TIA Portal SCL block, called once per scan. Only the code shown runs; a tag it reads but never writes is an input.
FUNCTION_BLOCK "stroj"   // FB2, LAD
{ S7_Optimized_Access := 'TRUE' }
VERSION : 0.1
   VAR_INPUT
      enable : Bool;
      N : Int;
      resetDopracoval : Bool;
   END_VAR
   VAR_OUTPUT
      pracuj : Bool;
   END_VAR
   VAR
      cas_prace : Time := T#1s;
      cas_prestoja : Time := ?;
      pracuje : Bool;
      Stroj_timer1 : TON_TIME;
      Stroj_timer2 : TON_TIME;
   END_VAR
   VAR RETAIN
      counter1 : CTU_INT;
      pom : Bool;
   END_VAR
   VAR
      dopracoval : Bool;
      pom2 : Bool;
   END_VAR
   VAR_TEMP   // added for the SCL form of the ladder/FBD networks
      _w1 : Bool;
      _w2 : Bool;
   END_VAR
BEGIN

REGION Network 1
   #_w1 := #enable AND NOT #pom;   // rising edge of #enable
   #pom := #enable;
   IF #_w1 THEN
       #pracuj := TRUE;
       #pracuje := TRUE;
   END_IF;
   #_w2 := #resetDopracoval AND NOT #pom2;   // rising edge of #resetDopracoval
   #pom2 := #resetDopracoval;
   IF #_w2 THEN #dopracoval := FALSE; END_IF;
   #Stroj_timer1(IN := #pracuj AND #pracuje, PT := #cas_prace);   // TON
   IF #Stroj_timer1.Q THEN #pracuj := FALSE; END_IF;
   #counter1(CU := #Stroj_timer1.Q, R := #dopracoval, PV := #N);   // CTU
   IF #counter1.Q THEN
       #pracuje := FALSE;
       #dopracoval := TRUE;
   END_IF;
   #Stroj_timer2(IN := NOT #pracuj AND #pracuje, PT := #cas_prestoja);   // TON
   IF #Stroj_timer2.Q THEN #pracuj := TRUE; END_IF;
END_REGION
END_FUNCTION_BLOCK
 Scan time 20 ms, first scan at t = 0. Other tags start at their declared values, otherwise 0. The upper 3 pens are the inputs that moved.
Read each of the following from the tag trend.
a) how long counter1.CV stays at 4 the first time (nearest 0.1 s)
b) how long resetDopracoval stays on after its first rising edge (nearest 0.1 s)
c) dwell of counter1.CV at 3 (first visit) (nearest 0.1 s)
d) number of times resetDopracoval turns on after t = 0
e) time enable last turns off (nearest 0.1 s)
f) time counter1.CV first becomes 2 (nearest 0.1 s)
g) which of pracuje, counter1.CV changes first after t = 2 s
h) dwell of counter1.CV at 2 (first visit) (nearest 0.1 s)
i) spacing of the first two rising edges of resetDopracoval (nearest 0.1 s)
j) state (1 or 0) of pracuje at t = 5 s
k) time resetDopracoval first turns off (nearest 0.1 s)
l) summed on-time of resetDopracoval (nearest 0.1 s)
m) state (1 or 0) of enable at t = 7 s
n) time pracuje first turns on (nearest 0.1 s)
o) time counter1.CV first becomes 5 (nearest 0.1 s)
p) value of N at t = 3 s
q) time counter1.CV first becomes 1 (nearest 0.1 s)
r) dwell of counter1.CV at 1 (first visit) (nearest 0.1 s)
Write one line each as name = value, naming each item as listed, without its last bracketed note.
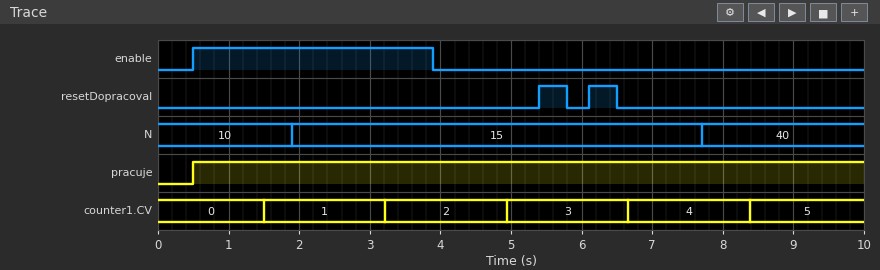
how long counter1.CV stays at 4 the first time = 1.7 s
how long resetDopracoval stays on after its first rising edge = 0.4 s
dwell of counter1.CV at 3 (first visit) = 1.7 s
number of times resetDopracoval turns on after t = 0 = 2
time enable last turns off = 3.9 s
time counter1.CV first becomes 2 = 3.2 s
which of pracuje, counter1.CV changes first after t = 2 s = counter1.CV
dwell of counter1.CV at 2 (first visit) = 1.7 s
spacing of the first two rising edges of resetDopracoval = 0.7 s
state (1 or 0) of pracuje at t = 5 s = 1
time resetDopracoval first turns off = 5.8 s
summed on-time of resetDopracoval = 0.8 s
state (1 or 0) of enable at t = 7 s = 0
time pracuje first turns on = 0.5 s
time counter1.CV first becomes 5 = 8.4 s
value of N at t = 3 s = 15
time counter1.CV first becomes 1 = 1.5 s
dwell of counter1.CV at 1 (first visit) = 1.7 s
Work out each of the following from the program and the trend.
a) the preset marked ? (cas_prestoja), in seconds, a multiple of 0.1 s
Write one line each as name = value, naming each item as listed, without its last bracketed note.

the preset marked ? (cas_prestoja), in seconds, a multiple of 0.1 s = 0.7 s
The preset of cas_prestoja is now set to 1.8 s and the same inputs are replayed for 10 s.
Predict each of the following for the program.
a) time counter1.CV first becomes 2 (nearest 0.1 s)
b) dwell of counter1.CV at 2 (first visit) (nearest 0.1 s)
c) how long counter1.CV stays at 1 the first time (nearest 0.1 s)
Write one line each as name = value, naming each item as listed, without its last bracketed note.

time counter1.CV first becomes 2 = 4.3 s
dwell of counter1.CV at 2 (first visit) = 2.8 s
how long counter1.CV stays at 1 the first time = 2.8 s
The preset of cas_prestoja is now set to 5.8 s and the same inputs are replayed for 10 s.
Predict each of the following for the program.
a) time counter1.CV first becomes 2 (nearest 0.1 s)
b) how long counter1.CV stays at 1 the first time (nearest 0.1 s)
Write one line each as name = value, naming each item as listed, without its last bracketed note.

time counter1.CV first becomes 2 = 8.3 s
how long counter1.CV stays at 1 the first time = 6.8 s
